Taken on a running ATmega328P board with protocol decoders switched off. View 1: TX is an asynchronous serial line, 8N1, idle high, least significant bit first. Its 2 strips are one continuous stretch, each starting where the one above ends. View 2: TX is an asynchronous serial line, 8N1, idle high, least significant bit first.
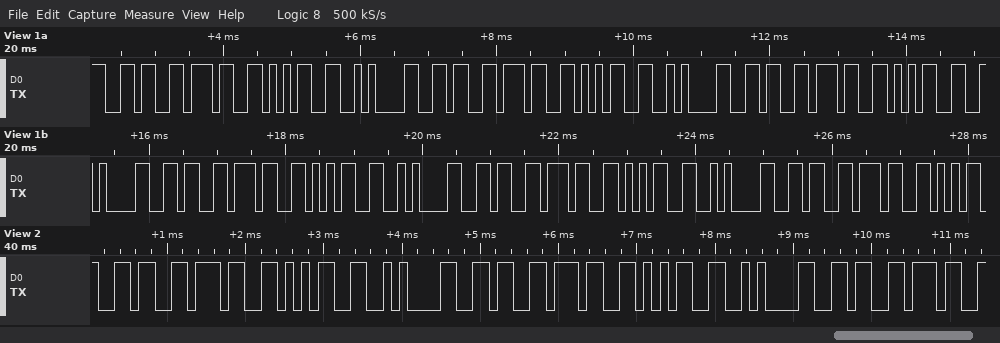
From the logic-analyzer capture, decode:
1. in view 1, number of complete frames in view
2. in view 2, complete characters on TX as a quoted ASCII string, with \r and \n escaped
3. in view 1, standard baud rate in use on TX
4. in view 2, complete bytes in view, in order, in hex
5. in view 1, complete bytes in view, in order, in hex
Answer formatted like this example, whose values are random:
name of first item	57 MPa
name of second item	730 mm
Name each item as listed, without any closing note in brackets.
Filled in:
in view 1, number of complete frames in view	22
in view 2, complete characters on TX as a quoted ASCII string, with \r and \n escaped	"675\n675\n67"
in view 1, standard baud rate in use on TX	9600 baud
in view 2, complete bytes in view, in order, in hex	0x36 0x37 0x35 0x0A 0x36 0x37 0x35 0x0A 0x36 0x37
in view 1, complete bytes in view, in order, in hex	36 37 35 0A 36 37 35 0A 36 37 35 0A 36 37 35 0A 36 37 35 0A 36 37
